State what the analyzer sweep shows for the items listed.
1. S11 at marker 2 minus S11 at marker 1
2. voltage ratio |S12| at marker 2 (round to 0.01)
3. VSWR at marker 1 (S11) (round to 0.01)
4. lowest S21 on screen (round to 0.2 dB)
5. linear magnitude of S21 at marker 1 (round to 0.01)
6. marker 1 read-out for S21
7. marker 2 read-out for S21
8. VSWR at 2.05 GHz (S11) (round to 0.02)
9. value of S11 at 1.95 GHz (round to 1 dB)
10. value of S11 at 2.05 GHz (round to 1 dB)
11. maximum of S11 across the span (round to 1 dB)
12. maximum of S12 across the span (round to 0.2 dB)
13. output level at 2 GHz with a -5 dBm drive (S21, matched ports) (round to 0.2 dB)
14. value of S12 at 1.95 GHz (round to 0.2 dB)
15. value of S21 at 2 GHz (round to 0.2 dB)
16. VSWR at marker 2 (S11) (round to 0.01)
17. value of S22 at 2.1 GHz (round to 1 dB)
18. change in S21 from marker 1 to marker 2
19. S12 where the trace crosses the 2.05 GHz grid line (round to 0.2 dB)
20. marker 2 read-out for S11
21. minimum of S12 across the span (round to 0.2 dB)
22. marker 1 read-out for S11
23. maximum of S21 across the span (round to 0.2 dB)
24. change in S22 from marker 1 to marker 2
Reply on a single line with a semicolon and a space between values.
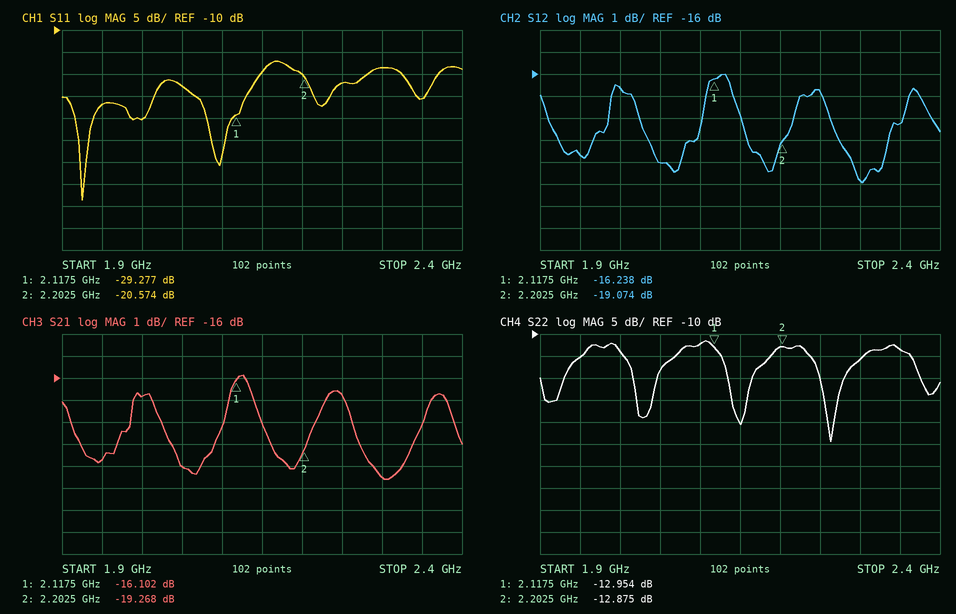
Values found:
8.703 dB; 0.11; 1.07; -20.6 dB; 0.16; -16.102 dB; -19.268 dB; 1.16; -27 dB; -23 dB; -17 dB; -16.0 dB; -21.8 dBm; -19.6 dB; -16.8 dB; 1.21; -12 dB; -3.166 dB; -20.0 dB; -20.574 dB; -21.0 dB; -29.277 dB; -15.8 dB; 0.079 dB
